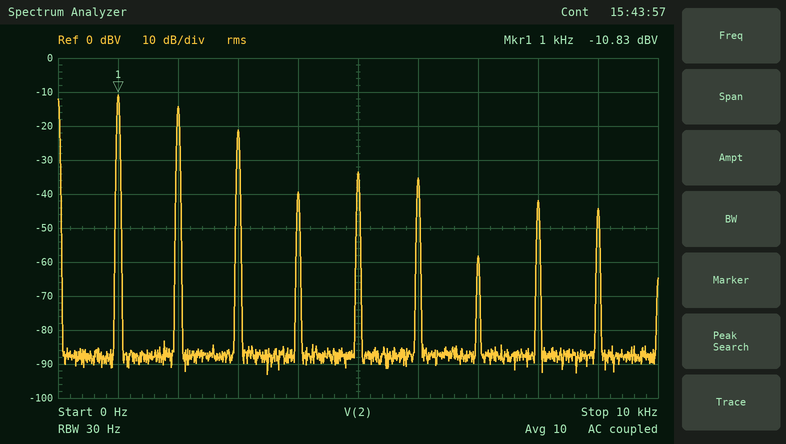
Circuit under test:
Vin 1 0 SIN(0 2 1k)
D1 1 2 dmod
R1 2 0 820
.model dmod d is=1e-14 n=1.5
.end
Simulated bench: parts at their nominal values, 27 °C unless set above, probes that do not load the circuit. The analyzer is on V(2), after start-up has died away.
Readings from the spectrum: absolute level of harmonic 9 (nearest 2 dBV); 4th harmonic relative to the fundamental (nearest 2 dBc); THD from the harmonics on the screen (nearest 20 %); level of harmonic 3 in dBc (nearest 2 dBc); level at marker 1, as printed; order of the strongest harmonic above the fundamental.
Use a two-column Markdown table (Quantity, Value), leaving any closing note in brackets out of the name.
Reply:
| Quantity | Value |
|---|---|
| absolute level of harmonic 9 | -44 dBV |
| 4th harmonic relative to the fundamental | -28 dBc |
| THD from the harmonics on the screen | 80 % |
| level of harmonic 3 in dBc | -10 dBc |
| level at marker 1, as printed | -10.83 dBV |
| order of the strongest harmonic above the fundamental | 2 |
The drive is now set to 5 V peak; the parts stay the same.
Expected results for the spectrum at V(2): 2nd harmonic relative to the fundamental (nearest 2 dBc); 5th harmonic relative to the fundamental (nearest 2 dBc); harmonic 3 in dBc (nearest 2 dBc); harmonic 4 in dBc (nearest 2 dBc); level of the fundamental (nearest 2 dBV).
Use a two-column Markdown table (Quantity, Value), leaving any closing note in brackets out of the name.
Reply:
| Quantity | Value |
|---|---|
| 2nd harmonic relative to the fundamental | -6 dBc |
| 5th harmonic relative to the fundamental | -26 dBc |
| harmonic 3 in dBc | -20 dBc |
| harmonic 4 in dBc | -22 dBc |
| level of the fundamental | 2 dBV |
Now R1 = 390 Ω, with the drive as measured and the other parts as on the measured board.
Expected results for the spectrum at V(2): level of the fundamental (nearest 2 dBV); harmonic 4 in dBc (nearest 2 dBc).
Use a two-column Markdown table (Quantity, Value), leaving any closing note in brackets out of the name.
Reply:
| Quantity | Value |
|---|---|
| level of the fundamental | -12 dBV |
| harmonic 4 in dBc | -26 dBc |
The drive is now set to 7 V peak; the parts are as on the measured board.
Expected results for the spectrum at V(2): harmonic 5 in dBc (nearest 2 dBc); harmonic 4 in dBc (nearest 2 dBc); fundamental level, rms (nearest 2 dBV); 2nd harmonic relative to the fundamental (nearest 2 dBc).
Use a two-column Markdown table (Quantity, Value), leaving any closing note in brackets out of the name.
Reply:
| Quantity | Value |
|---|---|
| harmonic 5 in dBc | -28 dBc |
| harmonic 4 in dBc | -22 dBc |
| fundamental level, rms | 6 dBV |
| 2nd harmonic relative to the fundamental | -6 dBc |
